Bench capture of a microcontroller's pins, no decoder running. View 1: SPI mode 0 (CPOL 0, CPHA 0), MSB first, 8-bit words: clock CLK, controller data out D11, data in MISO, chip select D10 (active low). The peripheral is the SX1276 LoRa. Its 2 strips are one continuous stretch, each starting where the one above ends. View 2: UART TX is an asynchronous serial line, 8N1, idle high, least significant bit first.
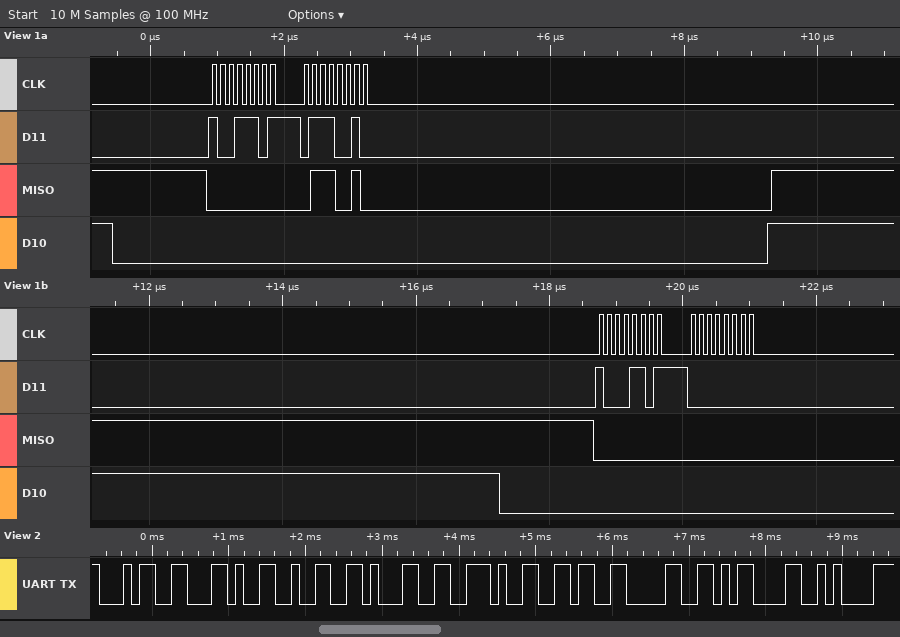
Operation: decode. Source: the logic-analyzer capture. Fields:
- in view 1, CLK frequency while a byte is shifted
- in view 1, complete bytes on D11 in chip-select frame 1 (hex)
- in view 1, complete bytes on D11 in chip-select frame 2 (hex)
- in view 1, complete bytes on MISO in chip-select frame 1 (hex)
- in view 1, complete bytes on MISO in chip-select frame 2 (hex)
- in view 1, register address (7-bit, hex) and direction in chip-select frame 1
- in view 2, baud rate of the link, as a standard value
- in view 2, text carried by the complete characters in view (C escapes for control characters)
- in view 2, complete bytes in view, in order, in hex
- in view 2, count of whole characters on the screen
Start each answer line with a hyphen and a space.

- 8 MHz
- 9D 72
- 8D 00
- 00 72
- 00 00
- 0x1D write
- 9600 baud
- "4,21.60\r\n"
- 34 2C 32 31 2E 36 30 0D 0A
- 9
